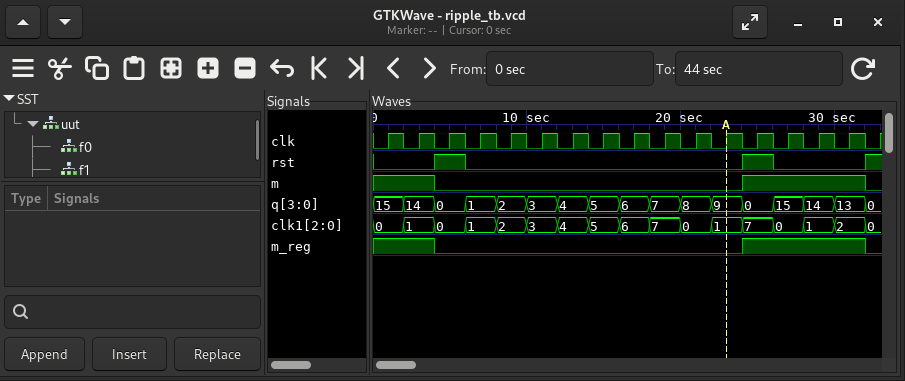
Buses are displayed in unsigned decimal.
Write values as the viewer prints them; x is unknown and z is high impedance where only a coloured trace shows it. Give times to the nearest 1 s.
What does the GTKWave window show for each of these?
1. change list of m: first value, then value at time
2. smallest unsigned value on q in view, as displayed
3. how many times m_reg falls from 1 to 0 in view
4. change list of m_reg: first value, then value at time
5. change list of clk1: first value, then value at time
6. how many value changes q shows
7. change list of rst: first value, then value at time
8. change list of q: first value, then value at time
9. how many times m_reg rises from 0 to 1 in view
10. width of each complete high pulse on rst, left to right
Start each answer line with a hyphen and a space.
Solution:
- 1, 0 at 4 s, 1 at 24 s, 0 at 32 s
- 0
- 2
- 1, 0 at 4 s, 1 at 24 s, 0 at 32 s
- 0, 1 at 2 s, 0 at 4 s, 1 at 6 s, 2 at 8 s, 3 at 10 s, 4 at 12 s, 5 at 14 s, 6 at 16 s, 7 at 18 s, 0 at 20 s, 1 at 22 s, 7 at 24 s, 0 at 26 s, 1 at 28 s, 2 at 30 s, 0 at 32 s
- 16
- 0, 1 at 4 s, 0 at 6 s, 1 at 24 s, 0 at 26 s, 1 at 32 s
- 15, 14 at 2 s, 0 at 4 s, 1 at 6 s, 2 at 8 s, 3 at 10 s, 4 at 12 s, 5 at 14 s, 6 at 16 s, 7 at 18 s, 8 at 20 s, 9 at 22 s, 0 at 24 s, 15 at 26 s, 14 at 28 s, 13 at 30 s, 0 at 32 s
- 1
- 2 s, 2 s
